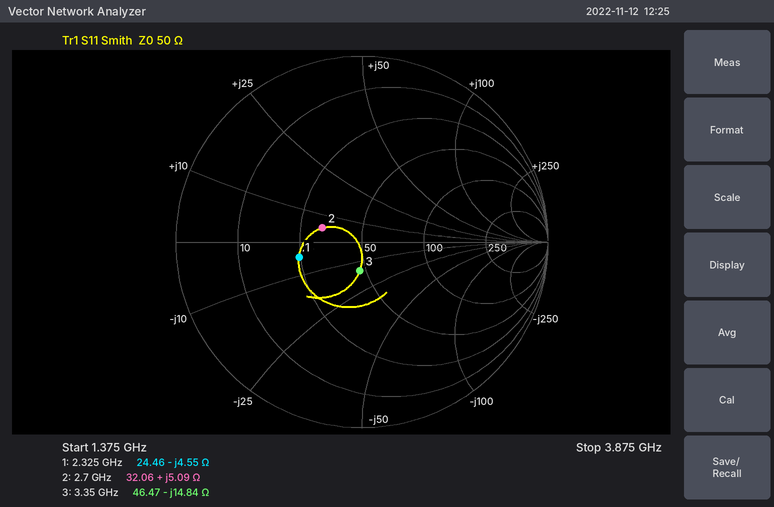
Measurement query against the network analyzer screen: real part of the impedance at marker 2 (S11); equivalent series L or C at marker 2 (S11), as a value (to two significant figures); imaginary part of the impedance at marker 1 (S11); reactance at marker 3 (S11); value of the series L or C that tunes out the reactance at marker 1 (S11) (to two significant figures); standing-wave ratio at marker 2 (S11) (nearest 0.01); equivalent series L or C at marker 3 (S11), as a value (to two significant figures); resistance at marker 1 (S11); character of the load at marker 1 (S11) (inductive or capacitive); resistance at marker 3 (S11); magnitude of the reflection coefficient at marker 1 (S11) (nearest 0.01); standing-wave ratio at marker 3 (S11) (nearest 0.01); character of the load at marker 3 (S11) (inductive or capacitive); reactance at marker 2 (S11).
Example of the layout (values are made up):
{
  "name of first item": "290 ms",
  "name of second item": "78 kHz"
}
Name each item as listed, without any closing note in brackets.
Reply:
{
  "real part of the impedance at marker 2": "32.06 Ω",
  "equivalent series L or C at marker 2 (S11), as a value": "300 pH",
  "imaginary part of the impedance at marker 1": "-4.55 Ω",
  "reactance at marker 3": "-14.84 Ω",
  "value of the series L or C that tunes out the reactance at marker 1 (S11)": "310 pH",
  "standing-wave ratio at marker 2 (S11)": "1.59",
  "equivalent series L or C at marker 3 (S11), as a value": "3.2 pF",
  "resistance at marker 1": "24.46 Ω",
  "character of the load at marker 1 (S11)": "capacitive",
  "resistance at marker 3": "46.47 Ω",
  "magnitude of the reflection coefficient at marker 1 (S11)": "0.35",
  "standing-wave ratio at marker 3 (S11)": "1.37",
  "character of the load at marker 3 (S11)": "capacitive",
  "reactance at marker 2": "+5.09 Ω"
}
